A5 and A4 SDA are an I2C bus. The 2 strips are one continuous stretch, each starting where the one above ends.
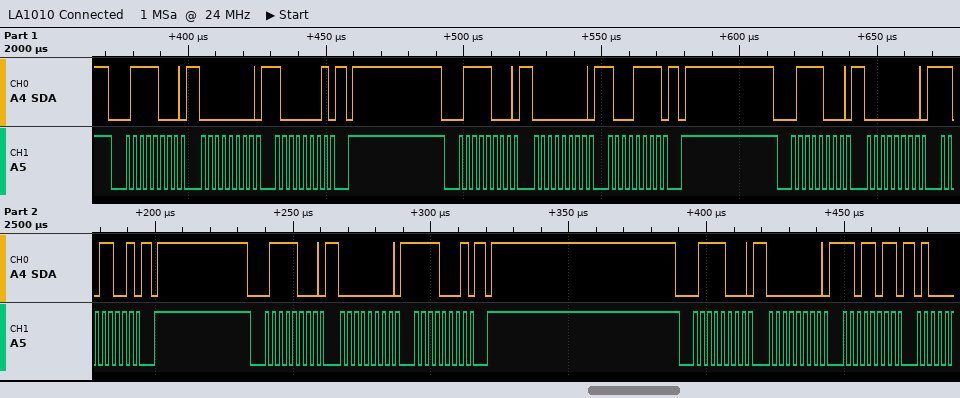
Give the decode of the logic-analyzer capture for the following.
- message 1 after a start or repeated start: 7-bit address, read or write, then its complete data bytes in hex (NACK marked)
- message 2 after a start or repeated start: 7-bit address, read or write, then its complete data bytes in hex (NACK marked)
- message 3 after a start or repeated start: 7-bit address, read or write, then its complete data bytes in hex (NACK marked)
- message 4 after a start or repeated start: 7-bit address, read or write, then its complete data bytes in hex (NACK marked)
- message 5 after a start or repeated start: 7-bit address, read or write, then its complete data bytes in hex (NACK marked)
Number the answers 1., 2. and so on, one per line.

1. 0x3C write: 00 81
2. 0x3C write: 00 8F
3. 0x3C write: 00 D9
4. 0x3C write: 00 F1
5. 0x3C write: 00 DB
